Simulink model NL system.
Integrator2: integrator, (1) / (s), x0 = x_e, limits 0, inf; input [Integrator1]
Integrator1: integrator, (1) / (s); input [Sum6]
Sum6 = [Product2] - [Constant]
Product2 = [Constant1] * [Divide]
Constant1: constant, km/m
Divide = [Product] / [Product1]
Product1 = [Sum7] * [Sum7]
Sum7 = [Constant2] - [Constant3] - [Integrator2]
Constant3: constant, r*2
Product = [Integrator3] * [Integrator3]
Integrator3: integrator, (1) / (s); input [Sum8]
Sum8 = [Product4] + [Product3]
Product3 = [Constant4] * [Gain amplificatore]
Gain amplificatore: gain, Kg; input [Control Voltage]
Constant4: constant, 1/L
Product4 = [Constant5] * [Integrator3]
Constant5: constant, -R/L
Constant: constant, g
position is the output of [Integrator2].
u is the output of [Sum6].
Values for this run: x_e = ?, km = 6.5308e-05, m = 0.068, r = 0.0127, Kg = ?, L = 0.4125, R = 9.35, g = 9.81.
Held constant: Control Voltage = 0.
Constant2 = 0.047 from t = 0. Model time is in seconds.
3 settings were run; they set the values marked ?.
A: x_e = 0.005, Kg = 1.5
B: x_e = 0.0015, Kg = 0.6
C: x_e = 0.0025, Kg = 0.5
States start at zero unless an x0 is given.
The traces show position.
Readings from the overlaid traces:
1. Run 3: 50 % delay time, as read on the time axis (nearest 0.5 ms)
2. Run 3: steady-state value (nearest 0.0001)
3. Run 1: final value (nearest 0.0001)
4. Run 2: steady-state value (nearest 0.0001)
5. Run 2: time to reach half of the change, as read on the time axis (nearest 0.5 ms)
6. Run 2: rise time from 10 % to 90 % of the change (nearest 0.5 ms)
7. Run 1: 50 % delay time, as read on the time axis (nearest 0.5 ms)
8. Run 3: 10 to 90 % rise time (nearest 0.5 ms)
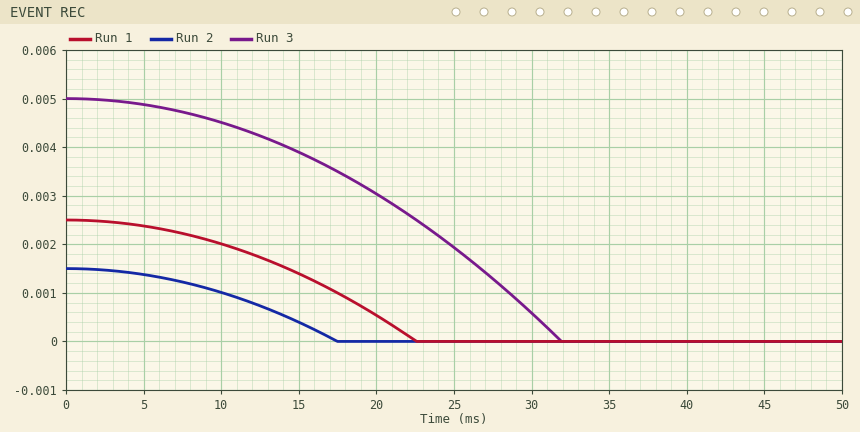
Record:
22.5 ms
0.0000
0.0000
0.0000
12.5 ms
11.0 ms
16.0 ms
20.0 ms
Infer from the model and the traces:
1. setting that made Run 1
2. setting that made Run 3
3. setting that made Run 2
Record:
C
A
B
